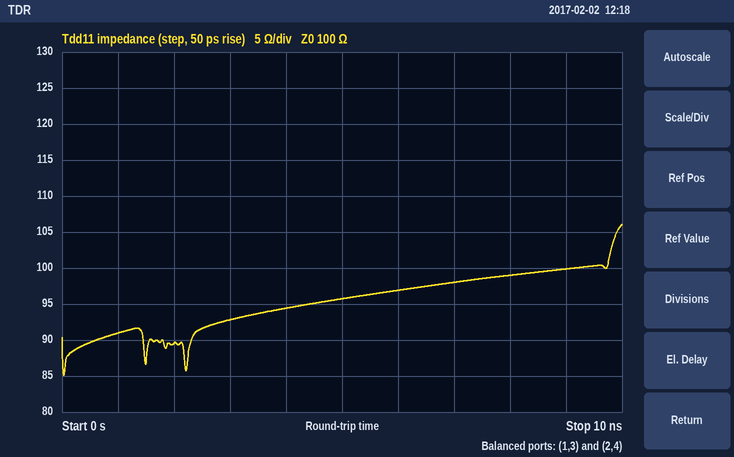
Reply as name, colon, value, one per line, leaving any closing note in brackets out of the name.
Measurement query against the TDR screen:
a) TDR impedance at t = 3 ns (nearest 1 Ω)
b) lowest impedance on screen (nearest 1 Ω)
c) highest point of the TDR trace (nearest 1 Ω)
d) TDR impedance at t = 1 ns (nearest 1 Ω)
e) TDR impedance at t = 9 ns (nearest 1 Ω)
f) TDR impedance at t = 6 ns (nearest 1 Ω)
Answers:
TDR impedance at t = 3 ns: 93 Ω
lowest impedance on screen: 85 Ω
highest point of the TDR trace: 106 Ω
TDR impedance at t = 1 ns: 91 Ω
TDR impedance at t = 9 ns: 100 Ω
TDR impedance at t = 6 ns: 97 Ω
